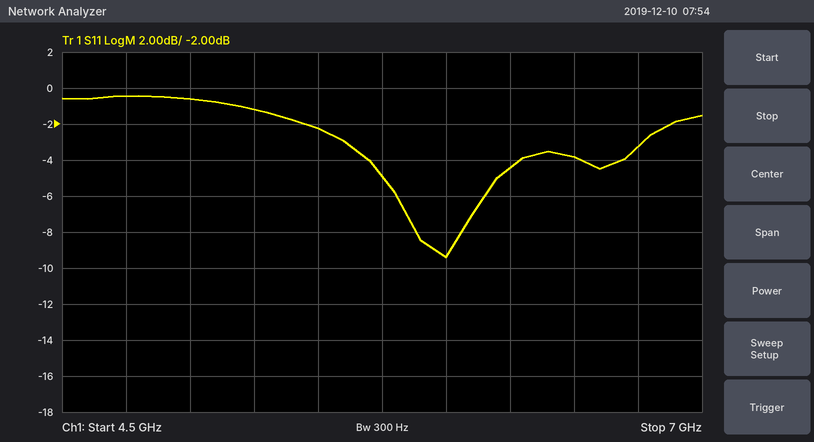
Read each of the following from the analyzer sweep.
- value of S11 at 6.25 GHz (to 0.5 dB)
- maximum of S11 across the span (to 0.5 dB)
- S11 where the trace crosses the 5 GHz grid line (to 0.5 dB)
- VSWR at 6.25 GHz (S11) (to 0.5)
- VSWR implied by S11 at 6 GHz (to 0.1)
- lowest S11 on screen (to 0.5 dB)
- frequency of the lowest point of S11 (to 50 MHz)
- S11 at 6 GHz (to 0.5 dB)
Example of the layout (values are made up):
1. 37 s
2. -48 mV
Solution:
1. -4.5 dB
2. -0.5 dB
3. -0.5 dB
4. 4.0
5. 2.0
6. -9.5 dB
7. 6.00 GHz
8. -9.5 dB
